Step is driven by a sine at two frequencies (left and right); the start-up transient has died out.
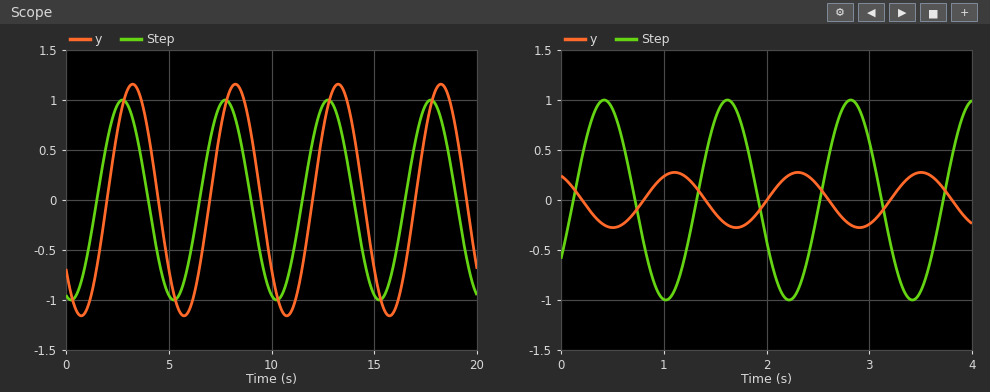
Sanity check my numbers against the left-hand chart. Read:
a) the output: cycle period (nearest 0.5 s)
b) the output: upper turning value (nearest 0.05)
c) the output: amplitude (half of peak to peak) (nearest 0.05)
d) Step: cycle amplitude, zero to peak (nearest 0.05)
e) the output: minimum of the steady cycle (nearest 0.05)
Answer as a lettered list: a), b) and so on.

a) 5.0 s
b) 1.15
c) 1.15
d) 1.00
e) -1.15
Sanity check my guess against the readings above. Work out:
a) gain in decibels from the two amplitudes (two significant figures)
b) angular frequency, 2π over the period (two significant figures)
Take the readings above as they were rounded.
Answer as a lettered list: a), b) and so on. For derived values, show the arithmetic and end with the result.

a) 20 log10(1.15 / 1) = 1.2 dB
b) 2π / 5 = 1.3 rad/s
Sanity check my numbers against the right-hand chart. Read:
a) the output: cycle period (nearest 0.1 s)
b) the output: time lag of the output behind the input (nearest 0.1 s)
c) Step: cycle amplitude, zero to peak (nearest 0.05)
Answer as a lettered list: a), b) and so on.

a) 1.2 s
b) 0.7 s
c) 1.00
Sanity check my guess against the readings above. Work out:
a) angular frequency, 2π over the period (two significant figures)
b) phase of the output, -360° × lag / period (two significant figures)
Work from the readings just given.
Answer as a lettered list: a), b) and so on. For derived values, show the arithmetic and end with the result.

a) 2π / 1.2 = 5.2 rad/s
b) -360 × 0.7 / 1.2 = -210°
